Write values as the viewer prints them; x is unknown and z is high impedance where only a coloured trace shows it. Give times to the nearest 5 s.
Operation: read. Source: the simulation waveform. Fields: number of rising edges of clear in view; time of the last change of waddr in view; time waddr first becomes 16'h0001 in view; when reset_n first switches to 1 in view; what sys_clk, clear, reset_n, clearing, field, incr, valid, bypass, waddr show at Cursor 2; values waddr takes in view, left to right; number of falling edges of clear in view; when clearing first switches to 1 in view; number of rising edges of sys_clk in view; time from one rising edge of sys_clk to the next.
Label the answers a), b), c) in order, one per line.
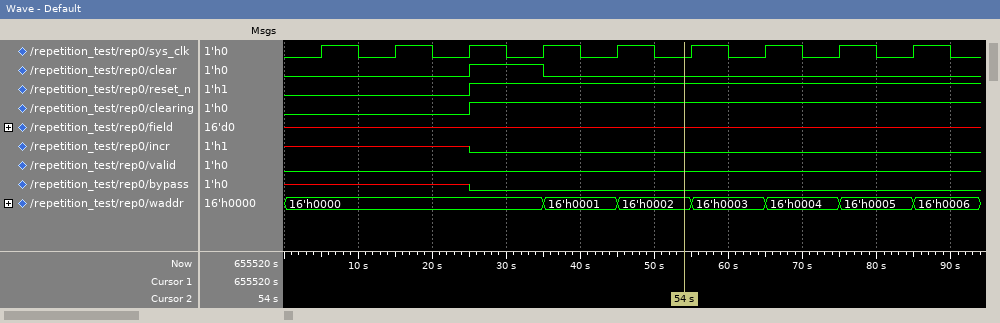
a) 1
b) 85 s
c) 35 s
d) 25 s
e) sys_clk=0, clear=0, reset_n=1, clearing=1, field=x, incr=0, valid=0, bypass=0, waddr=16'h0002
f) 16'h0000, 16'h0001, 16'h0002, 16'h0003, 16'h0004, 16'h0005, 16'h0006
g) 1
h) 25 s
i) 9
j) 10 s
